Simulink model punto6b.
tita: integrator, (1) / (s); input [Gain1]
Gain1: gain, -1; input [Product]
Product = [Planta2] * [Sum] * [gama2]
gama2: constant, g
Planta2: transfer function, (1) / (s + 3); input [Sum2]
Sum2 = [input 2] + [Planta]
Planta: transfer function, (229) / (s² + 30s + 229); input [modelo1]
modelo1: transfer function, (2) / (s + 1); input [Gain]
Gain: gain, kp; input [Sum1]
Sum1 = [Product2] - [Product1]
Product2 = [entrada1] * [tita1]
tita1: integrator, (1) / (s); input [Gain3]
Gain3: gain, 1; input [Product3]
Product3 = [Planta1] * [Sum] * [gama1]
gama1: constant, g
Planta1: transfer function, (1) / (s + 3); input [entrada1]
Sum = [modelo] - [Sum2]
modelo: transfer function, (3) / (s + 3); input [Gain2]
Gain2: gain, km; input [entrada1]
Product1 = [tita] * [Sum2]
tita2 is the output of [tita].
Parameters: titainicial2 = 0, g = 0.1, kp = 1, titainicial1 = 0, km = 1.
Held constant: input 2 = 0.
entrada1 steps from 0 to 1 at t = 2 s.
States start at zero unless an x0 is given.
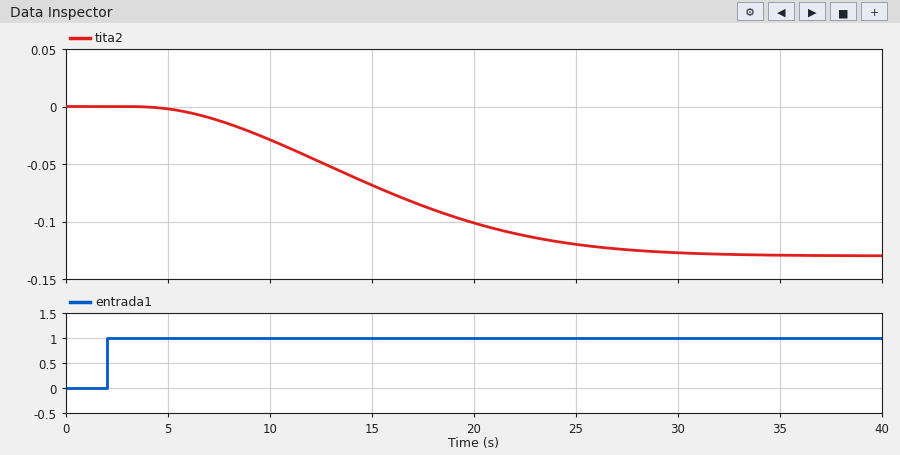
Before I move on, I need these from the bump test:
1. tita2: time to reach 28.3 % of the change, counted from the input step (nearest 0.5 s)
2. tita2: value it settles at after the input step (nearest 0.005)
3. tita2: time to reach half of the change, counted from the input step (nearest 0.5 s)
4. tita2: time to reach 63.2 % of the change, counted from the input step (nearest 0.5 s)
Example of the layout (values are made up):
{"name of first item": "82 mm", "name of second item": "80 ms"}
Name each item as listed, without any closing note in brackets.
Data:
{"tita2: time to reach 28.3 % of the change, counted from the input step": "9.0 s", "tita2: value it settles at after the input step": "-0.130", "tita2: time to reach half of the change, counted from the input step": "12.5 s", "tita2: time to reach 63.2 % of the change, counted from the input step": "15.0 s"}
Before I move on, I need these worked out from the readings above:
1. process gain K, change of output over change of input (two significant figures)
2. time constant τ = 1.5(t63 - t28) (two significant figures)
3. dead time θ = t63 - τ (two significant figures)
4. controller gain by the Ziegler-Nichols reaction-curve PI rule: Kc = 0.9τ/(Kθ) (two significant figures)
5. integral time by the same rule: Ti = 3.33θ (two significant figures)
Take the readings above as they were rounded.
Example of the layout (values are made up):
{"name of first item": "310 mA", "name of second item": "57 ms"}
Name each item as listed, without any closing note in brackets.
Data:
{"process gain K, change of output over change of input": "-0.13", "time constant τ = 1.5(t63 - t28)": "9.0 s", "dead time θ = t63 - τ": "6.0 s", "controller gain by the Ziegler-Nichols reaction-curve PI rule: Kc = 0.9τ/(Kθ)": "-10", "integral time by the same rule: Ti = 3.33θ": "20 s"}
